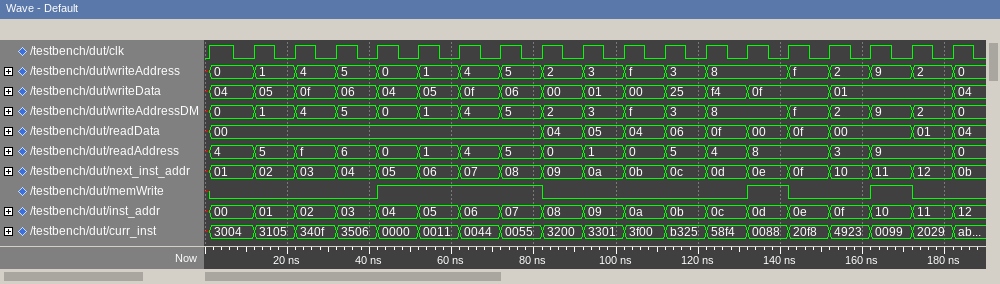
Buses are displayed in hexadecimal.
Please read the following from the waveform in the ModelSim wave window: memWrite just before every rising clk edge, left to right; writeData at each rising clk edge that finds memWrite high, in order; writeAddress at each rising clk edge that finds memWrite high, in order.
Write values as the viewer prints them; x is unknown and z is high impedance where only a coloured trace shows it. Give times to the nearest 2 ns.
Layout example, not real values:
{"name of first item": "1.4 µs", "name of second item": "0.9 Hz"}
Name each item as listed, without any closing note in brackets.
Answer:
{"memWrite just before every rising clk edge, left to right": "x 0 0 0 0 1 1 1 1 0 0 0 0 0 1 0 0 1 0", "writeData at each rising clk edge that finds memWrite high, in order": "04, 05, 0f, 06, 0f, 01", "writeAddress at each rising clk edge that finds memWrite high, in order": "0, 1, 4, 5, 8, 9"}
